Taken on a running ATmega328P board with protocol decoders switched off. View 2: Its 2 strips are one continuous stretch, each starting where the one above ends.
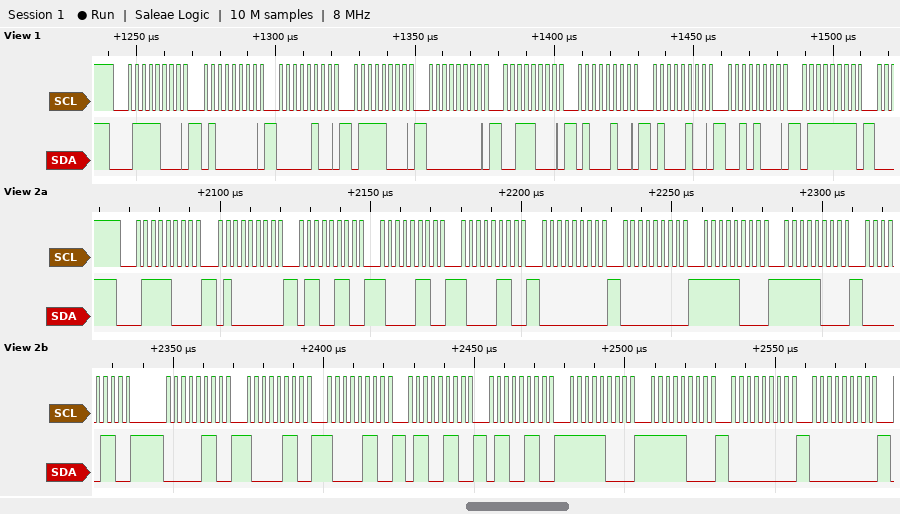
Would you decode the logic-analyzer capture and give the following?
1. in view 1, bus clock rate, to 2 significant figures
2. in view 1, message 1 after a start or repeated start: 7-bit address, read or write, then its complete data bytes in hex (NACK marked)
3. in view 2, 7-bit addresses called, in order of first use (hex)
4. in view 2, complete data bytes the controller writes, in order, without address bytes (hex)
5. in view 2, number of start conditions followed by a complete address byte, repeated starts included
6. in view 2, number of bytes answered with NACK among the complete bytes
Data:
400 kHz
0x3C write: 40 04 78 00 38 44 44 28 7F
0x3C
40 66 86 86 00 00 F8 F8 06 06 86 86 66 66 F8 F8 00 00
1
0
